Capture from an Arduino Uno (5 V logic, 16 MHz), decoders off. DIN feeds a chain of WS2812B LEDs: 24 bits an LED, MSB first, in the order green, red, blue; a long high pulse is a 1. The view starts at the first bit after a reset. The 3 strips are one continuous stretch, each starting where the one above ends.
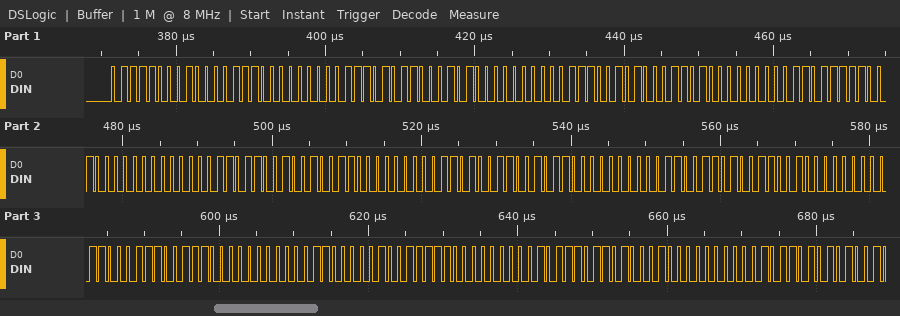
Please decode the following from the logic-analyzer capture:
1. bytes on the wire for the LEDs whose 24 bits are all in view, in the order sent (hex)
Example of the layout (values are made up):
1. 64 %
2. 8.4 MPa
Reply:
1. 78 87 00 75 8A 00 72 8D 00 6F 90 00 6C 93 00 69 96 00 66 99 00 63 9C 00 60 9F 00 5D A2 00
